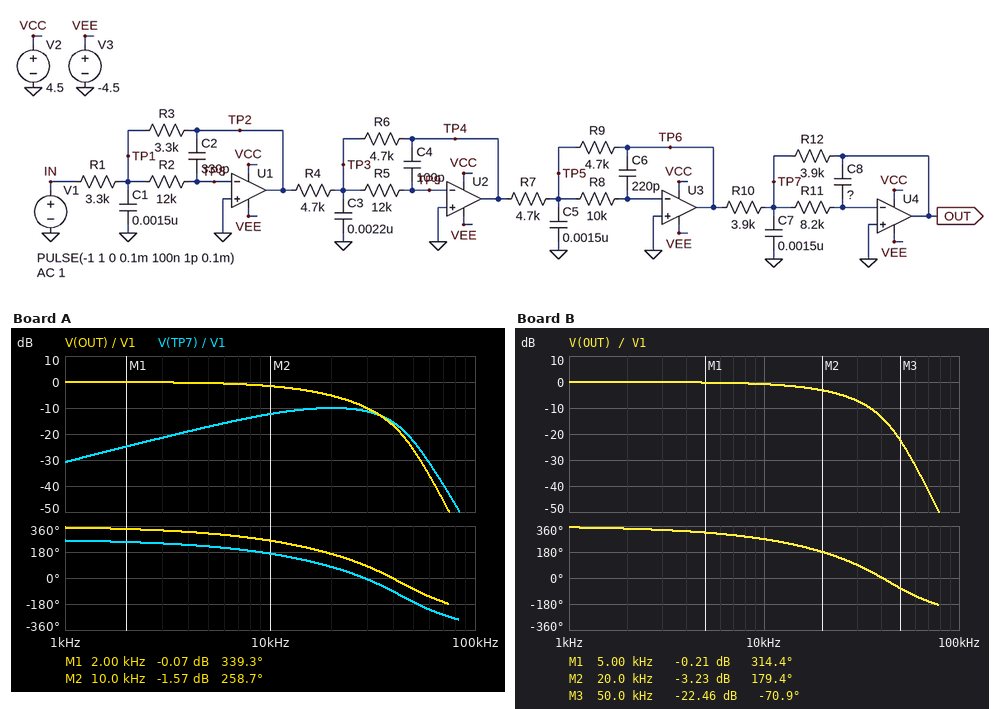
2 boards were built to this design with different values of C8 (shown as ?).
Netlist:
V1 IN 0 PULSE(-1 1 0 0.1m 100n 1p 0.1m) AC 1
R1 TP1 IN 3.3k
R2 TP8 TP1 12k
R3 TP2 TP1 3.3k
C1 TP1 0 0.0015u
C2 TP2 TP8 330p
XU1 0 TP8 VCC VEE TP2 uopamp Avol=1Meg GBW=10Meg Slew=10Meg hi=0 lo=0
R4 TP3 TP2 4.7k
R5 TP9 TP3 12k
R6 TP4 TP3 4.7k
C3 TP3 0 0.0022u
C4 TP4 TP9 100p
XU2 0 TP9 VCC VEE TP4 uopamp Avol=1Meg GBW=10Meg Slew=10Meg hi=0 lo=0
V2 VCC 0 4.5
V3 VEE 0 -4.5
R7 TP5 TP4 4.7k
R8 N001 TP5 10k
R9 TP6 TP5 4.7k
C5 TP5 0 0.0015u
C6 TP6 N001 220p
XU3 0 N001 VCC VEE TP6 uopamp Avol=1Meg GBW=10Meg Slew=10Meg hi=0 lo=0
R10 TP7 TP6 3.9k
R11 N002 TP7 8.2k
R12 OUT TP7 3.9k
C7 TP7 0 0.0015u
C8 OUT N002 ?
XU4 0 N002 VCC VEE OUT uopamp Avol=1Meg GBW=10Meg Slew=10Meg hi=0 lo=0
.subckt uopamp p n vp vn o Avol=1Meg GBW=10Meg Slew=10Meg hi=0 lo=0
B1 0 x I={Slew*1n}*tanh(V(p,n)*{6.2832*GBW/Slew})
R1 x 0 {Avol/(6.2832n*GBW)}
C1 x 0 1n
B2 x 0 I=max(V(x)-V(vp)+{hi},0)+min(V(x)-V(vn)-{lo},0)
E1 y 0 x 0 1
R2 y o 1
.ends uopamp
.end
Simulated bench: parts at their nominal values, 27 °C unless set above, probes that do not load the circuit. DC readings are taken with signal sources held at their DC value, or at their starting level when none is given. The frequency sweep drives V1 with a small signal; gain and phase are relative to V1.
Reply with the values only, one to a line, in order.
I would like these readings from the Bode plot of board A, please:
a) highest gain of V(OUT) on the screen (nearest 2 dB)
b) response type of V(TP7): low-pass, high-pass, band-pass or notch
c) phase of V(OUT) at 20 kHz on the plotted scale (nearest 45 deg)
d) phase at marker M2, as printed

0 dB
band-pass
180 deg
258.7 deg
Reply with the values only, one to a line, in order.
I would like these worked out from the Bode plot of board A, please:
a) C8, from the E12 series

560 pF
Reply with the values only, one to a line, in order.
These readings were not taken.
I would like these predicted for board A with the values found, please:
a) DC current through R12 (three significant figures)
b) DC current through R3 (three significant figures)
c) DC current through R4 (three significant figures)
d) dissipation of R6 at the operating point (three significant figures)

256 µA
303 µA
213 µA
213 µW
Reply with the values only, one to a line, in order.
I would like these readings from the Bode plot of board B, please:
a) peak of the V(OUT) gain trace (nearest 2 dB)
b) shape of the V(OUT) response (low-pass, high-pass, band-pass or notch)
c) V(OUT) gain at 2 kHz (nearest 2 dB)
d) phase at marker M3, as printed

0 dB
low-pass
0 dB
-70.9 deg
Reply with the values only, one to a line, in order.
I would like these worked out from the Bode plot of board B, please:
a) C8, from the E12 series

390 pF
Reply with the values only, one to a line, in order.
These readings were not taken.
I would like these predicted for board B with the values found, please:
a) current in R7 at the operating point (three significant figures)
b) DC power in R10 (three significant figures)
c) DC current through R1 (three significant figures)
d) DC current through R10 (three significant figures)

213 µA
256 µW
303 µA
256 µA
